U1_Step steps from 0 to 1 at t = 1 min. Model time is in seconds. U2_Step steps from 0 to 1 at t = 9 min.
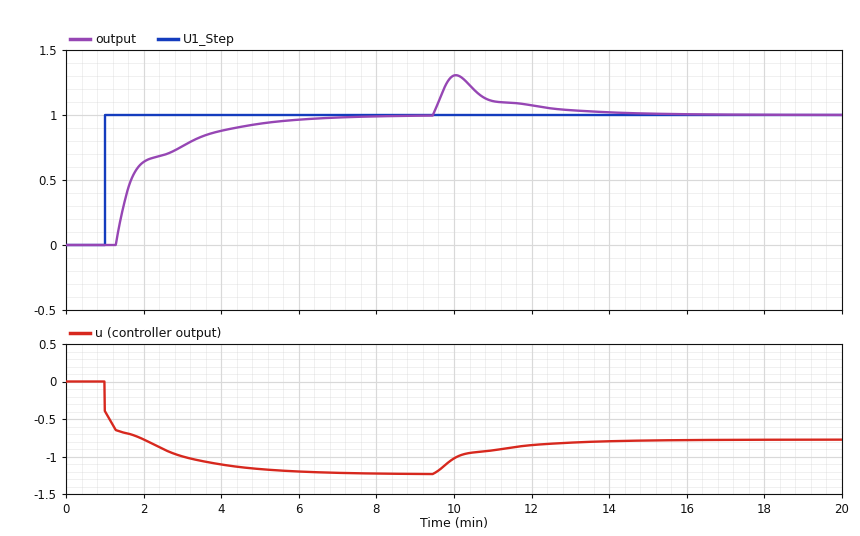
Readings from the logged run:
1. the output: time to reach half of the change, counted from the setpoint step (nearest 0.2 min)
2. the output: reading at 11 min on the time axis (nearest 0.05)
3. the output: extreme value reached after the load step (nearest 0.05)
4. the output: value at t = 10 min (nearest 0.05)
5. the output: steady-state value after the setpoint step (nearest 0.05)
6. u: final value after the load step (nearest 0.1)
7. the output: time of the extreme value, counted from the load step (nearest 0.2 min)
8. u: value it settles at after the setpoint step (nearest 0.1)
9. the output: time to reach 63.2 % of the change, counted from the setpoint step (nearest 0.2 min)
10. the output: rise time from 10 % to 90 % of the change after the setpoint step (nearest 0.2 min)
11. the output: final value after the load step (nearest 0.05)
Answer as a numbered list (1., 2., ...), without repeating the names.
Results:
1. 0.6 min
2. 1.10
3. 1.30
4. 1.30
5. 1.00
6. -0.8
7. 1.0 min
8. -1.2
9. 1.0 min
10. 3.0 min
11. 1.00
